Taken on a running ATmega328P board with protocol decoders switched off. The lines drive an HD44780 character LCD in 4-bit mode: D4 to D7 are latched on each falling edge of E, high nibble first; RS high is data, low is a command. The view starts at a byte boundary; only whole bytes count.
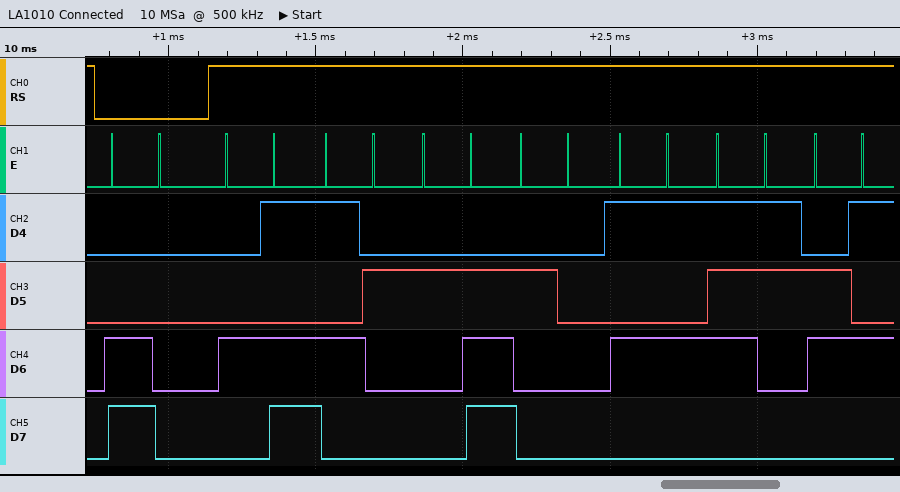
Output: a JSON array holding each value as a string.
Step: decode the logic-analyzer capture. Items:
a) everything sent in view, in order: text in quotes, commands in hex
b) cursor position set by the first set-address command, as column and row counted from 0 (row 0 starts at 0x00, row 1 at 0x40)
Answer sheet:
["0xC0 \"MR. Use\"", "column 0, row 1"]
